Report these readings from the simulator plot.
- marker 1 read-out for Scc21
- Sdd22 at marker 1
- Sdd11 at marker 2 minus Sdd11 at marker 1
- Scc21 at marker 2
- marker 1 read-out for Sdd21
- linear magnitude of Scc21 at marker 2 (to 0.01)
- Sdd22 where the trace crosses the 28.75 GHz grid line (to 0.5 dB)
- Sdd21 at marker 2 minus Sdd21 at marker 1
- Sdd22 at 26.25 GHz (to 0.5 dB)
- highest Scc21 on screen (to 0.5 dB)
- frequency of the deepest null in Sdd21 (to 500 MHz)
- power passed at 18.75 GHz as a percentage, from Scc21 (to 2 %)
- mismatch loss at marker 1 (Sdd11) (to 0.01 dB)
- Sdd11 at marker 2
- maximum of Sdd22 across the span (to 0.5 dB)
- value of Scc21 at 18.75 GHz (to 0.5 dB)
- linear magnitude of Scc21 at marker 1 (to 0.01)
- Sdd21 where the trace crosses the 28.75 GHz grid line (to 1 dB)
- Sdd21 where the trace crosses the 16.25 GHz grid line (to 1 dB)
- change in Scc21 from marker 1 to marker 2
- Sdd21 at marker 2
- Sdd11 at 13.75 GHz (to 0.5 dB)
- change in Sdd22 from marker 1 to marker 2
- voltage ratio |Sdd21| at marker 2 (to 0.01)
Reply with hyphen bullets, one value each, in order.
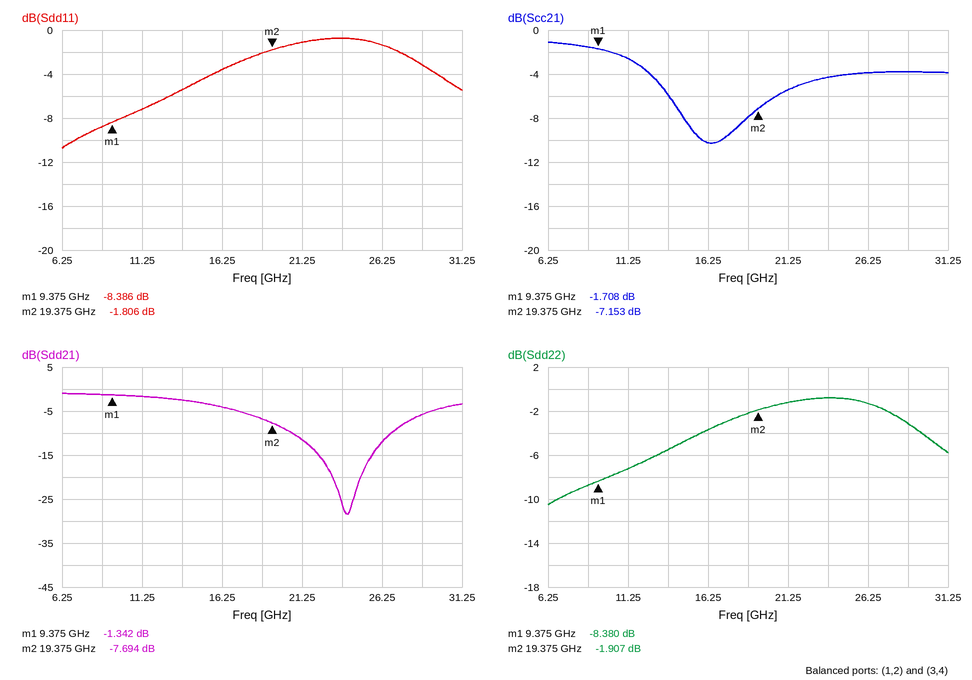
- -1.708 dB
- -8.380 dB
- 6.580 dB
- -7.153 dB
- -1.342 dB
- 0.44
- -3.0 dB
- -6.352 dB
- -1.5 dB
- -1.0 dB
- 24.0 GHz
- 16 %
- 0.68 dB
- -1.806 dB
- -1.0 dB
- -8.0 dB
- 0.82
- -6 dB
- -4 dB
- -5.445 dB
- -7.694 dB
- -5.5 dB
- 6.473 dB
- 0.41
